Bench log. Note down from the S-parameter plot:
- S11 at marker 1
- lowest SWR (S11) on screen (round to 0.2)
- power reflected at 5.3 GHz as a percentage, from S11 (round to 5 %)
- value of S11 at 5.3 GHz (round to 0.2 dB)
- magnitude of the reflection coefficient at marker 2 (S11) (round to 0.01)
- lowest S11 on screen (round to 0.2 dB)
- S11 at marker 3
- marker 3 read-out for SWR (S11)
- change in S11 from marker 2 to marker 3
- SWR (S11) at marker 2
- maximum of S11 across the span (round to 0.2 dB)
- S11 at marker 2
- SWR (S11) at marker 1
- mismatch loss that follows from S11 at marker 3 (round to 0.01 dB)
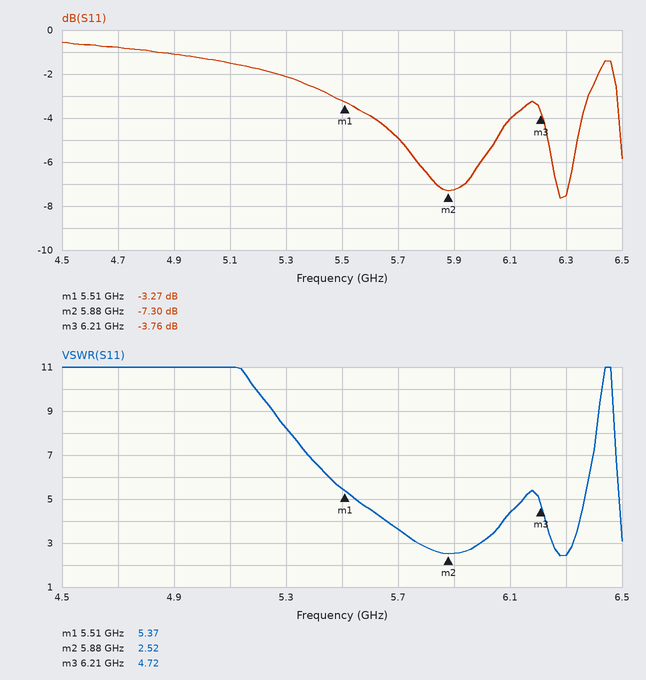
-3.27 dB
2.4
60 %
-2.2 dB
0.43
-7.6 dB
-3.76 dB
4.72
3.54 dB
2.52
-0.6 dB
-7.30 dB
5.37
2.37 dB
